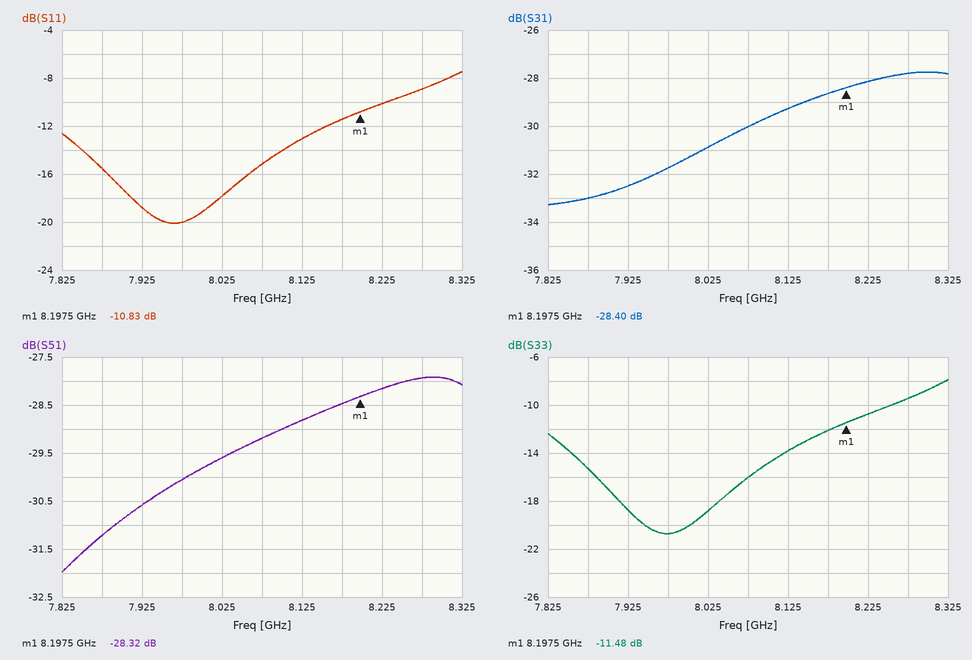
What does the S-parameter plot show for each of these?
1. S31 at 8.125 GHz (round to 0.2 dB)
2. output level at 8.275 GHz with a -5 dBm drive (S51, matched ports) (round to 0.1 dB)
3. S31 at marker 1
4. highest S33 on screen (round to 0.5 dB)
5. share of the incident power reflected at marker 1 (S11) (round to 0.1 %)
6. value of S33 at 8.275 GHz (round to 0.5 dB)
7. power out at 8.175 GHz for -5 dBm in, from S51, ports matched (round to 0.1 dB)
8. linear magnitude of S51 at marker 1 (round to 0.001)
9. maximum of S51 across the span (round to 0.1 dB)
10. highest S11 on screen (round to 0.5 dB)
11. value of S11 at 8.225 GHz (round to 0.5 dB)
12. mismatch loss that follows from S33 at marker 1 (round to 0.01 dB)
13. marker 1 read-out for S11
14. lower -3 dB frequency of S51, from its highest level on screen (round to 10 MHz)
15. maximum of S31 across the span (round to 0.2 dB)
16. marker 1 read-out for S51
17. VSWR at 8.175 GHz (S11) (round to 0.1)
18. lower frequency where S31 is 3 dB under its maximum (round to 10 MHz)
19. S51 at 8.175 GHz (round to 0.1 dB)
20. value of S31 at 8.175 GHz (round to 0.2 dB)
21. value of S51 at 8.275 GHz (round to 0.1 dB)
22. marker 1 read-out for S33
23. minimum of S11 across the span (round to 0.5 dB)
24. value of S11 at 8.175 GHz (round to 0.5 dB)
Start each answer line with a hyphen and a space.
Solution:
- -29.2 dB
- -32.9 dBm
- -28.40 dB
- -8.0 dB
- 8.3 %
- -9.5 dB
- -33.5 dBm
- 0.038
- -27.9 dB
- -7.5 dB
- -10.0 dB
- 0.32 dB
- -10.83 dB
- 7.90 GHz
- -27.8 dB
- -28.32 dB
- 1.7
- 8.03 GHz
- -28.5 dB
- -28.6 dB
- -27.9 dB
- -11.48 dB
- -20.0 dB
- -11.5 dB
